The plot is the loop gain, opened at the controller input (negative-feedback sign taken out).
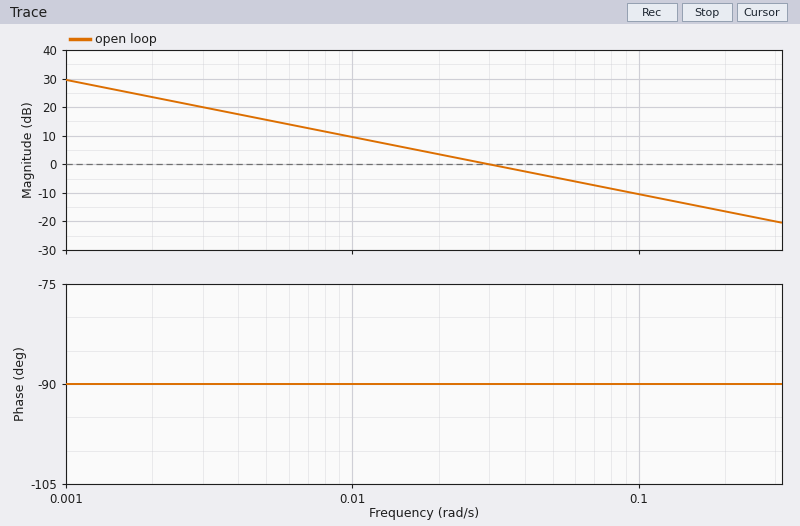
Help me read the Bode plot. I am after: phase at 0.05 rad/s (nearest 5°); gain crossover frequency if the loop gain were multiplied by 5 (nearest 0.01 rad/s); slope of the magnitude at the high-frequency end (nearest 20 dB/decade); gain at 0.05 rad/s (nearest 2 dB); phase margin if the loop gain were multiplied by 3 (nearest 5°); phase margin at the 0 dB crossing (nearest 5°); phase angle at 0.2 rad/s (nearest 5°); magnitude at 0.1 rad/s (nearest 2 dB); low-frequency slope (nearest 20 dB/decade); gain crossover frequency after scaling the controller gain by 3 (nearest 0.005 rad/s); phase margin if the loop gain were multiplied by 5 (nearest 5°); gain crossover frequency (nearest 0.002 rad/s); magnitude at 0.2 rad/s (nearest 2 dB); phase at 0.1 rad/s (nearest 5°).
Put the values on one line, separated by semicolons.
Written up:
-90°; 0.15 rad/s; -20 dB/decade; -4 dB; 90°; 90°; -90°; -10 dB; -20 dB/decade; 0.090 rad/s; 90°; 0.030 rad/s; -16 dB; -90°
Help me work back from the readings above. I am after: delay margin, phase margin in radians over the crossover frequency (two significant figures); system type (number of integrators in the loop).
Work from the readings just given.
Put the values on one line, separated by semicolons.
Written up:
52 s; 1
